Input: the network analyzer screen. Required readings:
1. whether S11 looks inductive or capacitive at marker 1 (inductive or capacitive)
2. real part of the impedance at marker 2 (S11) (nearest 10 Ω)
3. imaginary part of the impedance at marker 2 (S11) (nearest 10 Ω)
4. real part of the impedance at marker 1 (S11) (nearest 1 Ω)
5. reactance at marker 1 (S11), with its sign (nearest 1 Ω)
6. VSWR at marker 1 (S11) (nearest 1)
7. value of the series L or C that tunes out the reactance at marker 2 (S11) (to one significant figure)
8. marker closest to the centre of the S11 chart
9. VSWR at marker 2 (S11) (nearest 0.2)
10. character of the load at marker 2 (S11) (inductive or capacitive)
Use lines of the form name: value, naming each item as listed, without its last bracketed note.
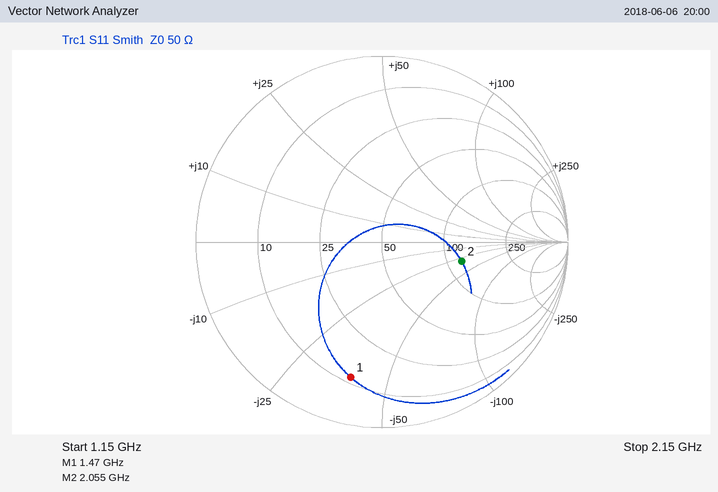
whether S11 looks inductive or capacitive at marker 1: capacitive
real part of the impedance at marker 2 (S11): 120 Ω
imaginary part of the impedance at marker 2 (S11): -30 Ω
real part of the impedance at marker 1 (S11): 12 Ω
reactance at marker 1 (S11), with its sign: -38 Ω
VSWR at marker 1 (S11): 7
value of the series L or C that tunes out the reactance at marker 2 (S11): 2 nH
marker closest to the centre of the S11 chart: marker 2
VSWR at marker 2 (S11): 2.6
character of the load at marker 2 (S11): capacitive
